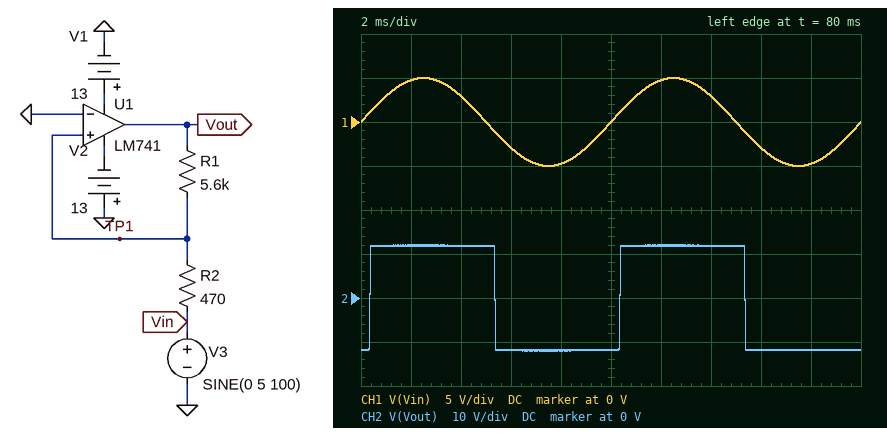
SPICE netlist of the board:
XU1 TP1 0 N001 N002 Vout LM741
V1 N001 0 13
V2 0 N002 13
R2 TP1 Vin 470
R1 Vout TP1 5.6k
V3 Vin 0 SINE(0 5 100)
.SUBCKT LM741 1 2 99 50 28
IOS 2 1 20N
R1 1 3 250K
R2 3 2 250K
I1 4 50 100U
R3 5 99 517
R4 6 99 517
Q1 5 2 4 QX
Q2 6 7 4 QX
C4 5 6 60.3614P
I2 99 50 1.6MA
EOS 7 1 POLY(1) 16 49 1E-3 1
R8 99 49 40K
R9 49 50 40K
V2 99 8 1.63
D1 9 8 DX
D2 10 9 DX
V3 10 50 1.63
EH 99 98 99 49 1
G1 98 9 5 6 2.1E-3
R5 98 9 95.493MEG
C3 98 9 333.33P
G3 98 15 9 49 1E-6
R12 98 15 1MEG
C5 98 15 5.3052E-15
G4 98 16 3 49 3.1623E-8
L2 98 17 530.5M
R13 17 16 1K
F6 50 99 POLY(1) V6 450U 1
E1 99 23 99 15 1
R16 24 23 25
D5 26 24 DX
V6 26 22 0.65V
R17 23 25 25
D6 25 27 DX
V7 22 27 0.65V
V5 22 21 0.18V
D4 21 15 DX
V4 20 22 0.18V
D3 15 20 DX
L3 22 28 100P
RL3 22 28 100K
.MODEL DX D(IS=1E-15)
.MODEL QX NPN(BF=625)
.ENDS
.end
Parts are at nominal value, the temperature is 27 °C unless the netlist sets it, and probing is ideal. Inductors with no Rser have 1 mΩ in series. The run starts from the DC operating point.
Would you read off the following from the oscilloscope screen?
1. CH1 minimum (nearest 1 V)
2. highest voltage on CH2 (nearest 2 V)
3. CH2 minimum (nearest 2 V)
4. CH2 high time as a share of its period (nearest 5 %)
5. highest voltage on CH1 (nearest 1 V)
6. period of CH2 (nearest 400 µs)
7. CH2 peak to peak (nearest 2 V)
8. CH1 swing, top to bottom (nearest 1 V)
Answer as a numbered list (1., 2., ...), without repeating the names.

1. -5 V
2. 12 V
3. -12 V
4. 50 %
5. 5 V
6. 10.0 ms
7. 24 V
8. 10 V
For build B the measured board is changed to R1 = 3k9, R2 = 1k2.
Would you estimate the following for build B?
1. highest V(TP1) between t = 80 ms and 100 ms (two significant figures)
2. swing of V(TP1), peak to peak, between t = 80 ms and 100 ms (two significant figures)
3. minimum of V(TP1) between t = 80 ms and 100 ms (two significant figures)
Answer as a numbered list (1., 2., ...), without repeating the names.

1. 6.6 V
2. 13 V
3. -6.6 V
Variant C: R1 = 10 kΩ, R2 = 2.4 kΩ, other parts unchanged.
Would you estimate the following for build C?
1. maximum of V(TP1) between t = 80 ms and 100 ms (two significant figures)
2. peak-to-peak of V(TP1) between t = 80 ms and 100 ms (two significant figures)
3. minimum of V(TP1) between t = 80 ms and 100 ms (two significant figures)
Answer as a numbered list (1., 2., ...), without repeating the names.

1. 6.3 V
2. 13 V
3. -6.3 V
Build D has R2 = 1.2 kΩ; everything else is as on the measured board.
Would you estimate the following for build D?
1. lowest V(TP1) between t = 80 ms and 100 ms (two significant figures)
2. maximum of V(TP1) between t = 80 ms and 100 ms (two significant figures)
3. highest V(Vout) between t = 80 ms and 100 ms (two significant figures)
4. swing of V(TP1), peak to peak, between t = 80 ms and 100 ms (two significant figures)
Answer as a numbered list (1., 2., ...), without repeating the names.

1. -6.2 V
2. 6.2 V
3. 12 V
4. 12 V
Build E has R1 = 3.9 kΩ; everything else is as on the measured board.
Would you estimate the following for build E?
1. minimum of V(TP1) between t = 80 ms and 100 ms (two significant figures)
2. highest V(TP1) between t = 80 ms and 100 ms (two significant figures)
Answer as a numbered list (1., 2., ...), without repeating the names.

1. -5.7 V
2. 5.7 V
